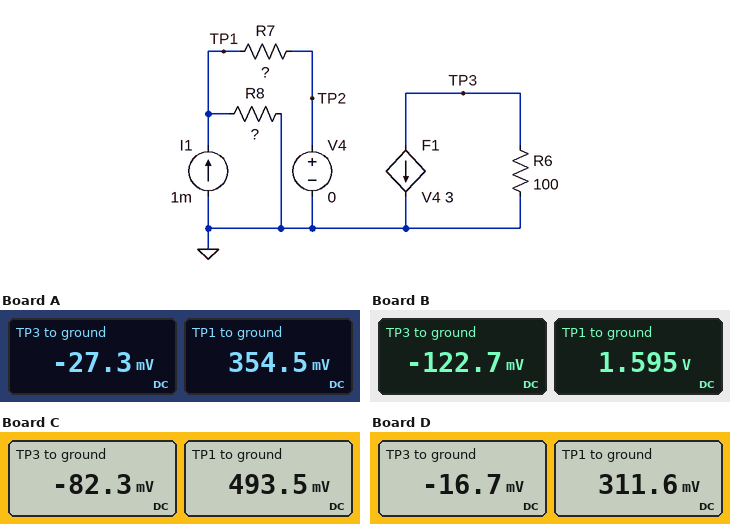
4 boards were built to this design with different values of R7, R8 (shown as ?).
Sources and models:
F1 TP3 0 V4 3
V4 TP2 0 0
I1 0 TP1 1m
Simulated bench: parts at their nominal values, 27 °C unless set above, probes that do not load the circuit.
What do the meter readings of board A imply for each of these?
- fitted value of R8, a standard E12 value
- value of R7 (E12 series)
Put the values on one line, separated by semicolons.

390 Ω; 3.9 kΩ
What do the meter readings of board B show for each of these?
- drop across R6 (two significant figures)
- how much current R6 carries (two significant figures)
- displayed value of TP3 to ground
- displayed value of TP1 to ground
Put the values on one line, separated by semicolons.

120 mV; 1.2 mA; -122.7 mV; 1.595 V
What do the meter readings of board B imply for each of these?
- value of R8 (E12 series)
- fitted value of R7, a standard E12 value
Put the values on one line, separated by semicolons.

2.7 kΩ; 3.9 kΩ
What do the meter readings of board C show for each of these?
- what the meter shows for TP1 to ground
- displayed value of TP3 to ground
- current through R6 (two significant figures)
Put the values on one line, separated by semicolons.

493.5 mV; -82.3 mV; 820 µA
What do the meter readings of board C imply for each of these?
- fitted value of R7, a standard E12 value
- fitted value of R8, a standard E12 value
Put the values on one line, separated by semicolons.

1.8 kΩ; 680 Ω
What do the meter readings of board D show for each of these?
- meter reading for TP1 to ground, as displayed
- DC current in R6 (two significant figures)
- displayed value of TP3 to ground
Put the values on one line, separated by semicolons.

311.6 mV; 170 µA; -16.7 mV
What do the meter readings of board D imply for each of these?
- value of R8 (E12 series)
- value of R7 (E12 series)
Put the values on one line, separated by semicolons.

330 Ω; 5.6 kΩ
